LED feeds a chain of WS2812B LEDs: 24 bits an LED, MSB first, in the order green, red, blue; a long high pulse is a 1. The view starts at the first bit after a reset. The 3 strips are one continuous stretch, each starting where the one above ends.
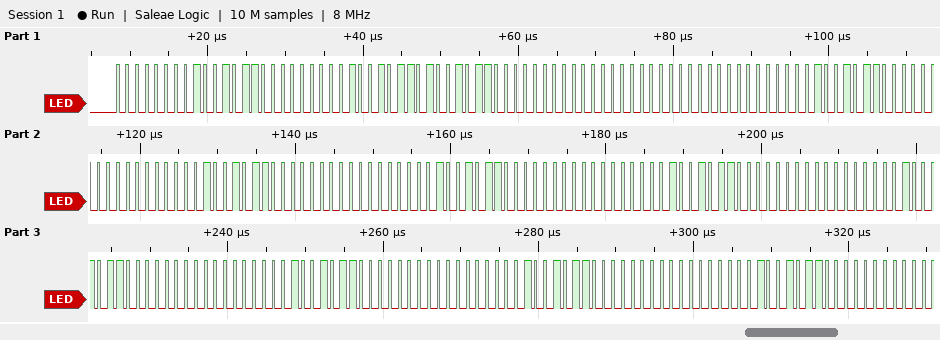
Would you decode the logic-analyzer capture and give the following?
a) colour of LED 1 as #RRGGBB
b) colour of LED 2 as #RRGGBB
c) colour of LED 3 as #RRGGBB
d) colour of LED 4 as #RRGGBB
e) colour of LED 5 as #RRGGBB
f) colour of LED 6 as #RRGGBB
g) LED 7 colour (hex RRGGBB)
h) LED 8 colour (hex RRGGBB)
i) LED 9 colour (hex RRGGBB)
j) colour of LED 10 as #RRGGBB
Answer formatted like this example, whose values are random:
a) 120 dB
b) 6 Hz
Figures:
a) #960000
b) #969600
c) #000000
d) #009600
e) #009600
f) #009600
g) #009600
h) #009600
i) #009600
j) #009600
